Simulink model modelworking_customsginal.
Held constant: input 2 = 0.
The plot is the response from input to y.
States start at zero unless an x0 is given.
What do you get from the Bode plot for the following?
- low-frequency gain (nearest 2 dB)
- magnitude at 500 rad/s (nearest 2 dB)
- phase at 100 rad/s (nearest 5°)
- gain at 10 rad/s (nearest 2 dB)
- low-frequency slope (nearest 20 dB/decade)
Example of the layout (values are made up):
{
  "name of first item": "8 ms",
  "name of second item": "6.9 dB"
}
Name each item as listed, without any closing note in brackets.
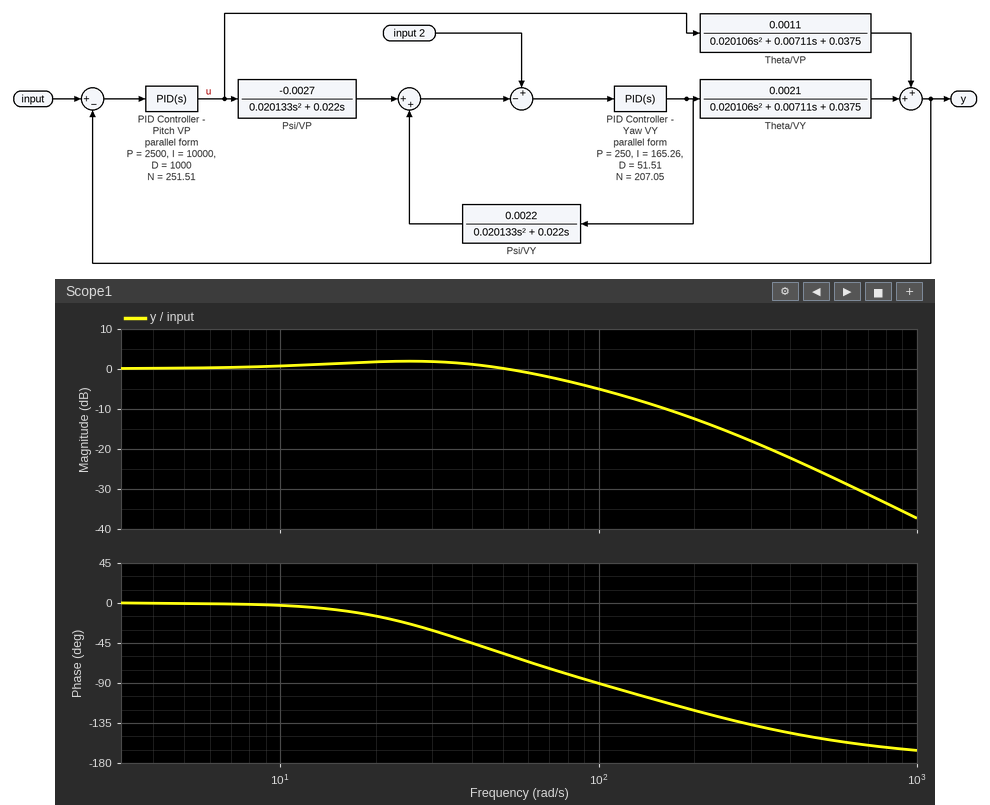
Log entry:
{
  "low-frequency gain": "0 dB",
  "magnitude at 500 rad/s": "-26 dB",
  "phase at 100 rad/s": "-90°",
  "gain at 10 rad/s": "0 dB",
  "low-frequency slope": "0 dB/decade"
}
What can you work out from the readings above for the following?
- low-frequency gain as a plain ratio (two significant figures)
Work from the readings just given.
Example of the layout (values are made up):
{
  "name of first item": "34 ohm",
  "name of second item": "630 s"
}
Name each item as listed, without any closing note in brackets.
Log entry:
{
  "low-frequency gain as a plain ratio": "1.0"
}
